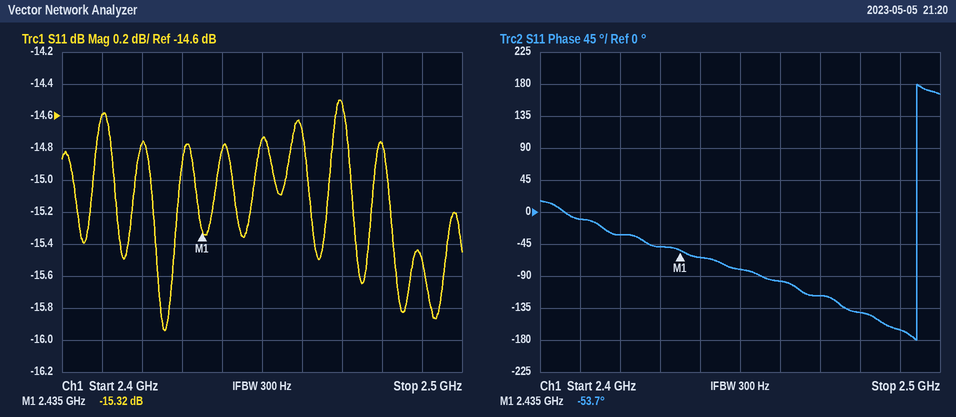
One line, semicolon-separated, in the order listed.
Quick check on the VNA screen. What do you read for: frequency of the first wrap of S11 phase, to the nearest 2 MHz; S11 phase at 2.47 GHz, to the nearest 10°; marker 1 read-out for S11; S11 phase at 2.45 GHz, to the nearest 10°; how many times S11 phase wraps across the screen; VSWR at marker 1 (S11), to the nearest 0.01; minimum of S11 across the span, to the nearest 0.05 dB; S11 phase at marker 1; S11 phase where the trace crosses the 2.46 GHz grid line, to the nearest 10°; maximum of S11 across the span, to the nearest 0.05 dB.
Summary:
2.494 GHz; -120°; -15.32 dB; -80°; 1; 1.41; -15.95 dB; -53.7°; -100°; -14.50 dB
